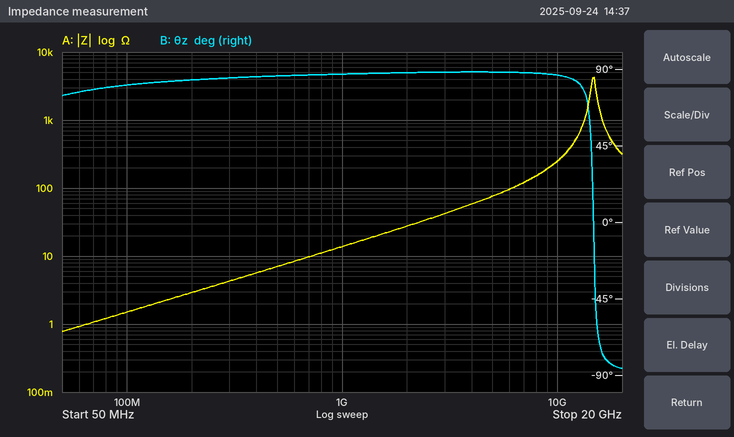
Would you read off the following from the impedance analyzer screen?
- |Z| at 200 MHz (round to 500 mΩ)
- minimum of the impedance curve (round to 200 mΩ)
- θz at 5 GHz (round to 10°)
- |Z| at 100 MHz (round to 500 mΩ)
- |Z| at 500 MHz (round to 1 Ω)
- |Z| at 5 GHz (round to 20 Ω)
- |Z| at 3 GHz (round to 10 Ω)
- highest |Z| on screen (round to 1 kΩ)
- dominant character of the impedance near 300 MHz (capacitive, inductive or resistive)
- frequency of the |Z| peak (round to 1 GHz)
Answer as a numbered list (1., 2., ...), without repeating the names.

1. 3.0 Ω
2. 800 mΩ
3. 90°
4. 1.5 Ω
5. 7 Ω
6. 80 Ω
7. 40 Ω
8. 4 kΩ
9. inductive
10. 15 GHz
